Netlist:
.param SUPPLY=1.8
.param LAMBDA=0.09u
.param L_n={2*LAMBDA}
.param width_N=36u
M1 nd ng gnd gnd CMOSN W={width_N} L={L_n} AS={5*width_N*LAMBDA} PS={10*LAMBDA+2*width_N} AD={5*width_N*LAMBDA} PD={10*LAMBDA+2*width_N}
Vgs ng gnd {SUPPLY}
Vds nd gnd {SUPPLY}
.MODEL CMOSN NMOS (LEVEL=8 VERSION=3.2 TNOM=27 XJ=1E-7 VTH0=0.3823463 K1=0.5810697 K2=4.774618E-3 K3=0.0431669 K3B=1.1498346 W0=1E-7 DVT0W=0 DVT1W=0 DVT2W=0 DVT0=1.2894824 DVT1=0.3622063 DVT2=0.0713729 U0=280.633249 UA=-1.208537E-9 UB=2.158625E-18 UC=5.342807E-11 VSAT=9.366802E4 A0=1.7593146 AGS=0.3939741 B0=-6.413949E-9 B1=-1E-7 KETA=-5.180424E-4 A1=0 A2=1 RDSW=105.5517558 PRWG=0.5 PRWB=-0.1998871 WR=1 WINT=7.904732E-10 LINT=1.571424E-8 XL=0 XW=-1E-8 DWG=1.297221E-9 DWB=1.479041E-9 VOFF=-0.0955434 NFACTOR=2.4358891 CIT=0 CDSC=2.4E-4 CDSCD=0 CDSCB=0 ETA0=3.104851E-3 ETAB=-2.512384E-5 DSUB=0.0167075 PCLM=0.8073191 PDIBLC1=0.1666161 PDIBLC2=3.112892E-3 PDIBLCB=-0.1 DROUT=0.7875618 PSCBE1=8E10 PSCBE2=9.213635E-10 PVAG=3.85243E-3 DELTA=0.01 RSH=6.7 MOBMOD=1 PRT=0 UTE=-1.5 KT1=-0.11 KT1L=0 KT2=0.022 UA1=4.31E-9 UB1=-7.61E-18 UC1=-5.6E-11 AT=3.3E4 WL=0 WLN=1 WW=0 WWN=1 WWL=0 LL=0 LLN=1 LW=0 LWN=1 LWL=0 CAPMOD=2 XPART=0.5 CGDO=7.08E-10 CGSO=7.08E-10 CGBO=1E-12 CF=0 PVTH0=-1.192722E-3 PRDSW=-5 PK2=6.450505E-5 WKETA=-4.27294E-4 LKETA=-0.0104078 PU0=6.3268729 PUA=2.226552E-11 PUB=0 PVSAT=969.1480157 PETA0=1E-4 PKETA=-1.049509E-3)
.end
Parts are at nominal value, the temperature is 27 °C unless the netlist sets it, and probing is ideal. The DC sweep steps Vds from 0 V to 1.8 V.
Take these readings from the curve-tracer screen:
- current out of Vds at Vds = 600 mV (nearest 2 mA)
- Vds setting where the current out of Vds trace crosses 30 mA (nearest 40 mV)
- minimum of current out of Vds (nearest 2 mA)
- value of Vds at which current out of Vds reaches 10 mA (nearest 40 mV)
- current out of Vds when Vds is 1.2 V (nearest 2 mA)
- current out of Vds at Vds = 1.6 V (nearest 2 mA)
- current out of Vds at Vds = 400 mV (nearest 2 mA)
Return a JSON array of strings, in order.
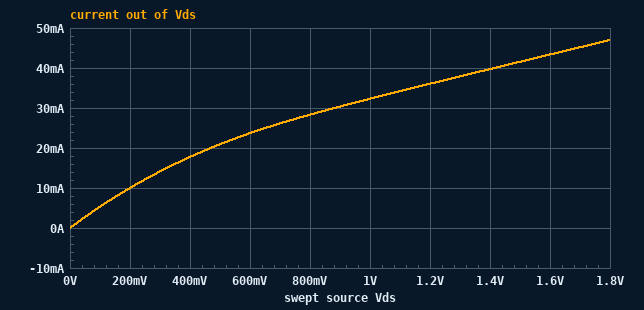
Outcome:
["24 mA", "880 mV", "0 A", "200 mV", "36 mA", "44 mA", "18 mA"]
